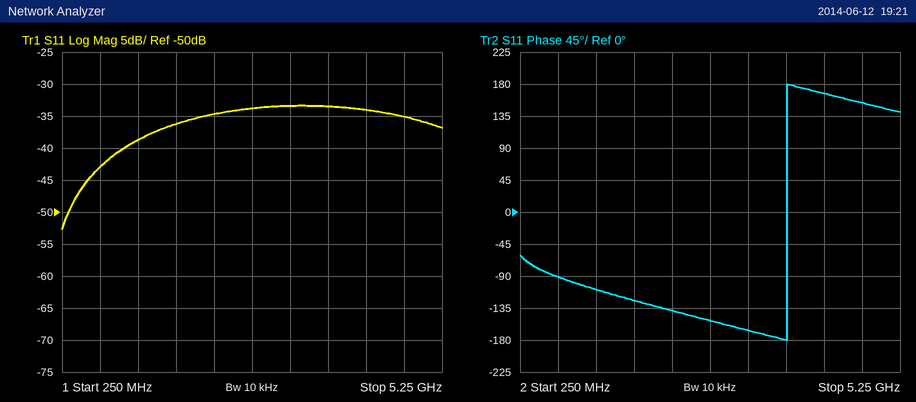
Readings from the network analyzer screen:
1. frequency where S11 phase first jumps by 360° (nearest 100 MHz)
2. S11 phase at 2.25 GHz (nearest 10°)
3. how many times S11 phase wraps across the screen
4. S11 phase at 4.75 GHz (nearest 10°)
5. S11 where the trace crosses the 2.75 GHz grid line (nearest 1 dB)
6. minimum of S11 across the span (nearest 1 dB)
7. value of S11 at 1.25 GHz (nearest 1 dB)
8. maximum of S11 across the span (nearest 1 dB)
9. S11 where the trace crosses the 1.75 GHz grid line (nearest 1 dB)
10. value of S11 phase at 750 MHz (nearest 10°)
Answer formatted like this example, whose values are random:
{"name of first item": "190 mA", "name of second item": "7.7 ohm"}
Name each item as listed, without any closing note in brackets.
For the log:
{"frequency where S11 phase first jumps by 360°": "3.8 GHz", "S11 phase at 2.25 GHz": "-140°", "how many times S11 phase wraps across the screen": "1", "S11 phase at 4.75 GHz": "150°", "S11 where the trace crosses the 2.75 GHz grid line": "-34 dB", "minimum of S11 across the span": "-53 dB", "value of S11 at 1.25 GHz": "-39 dB", "maximum of S11 across the span": "-33 dB", "S11 where the trace crosses the 1.75 GHz grid line": "-36 dB", "value of S11 phase at 750 MHz": "-90°"}
